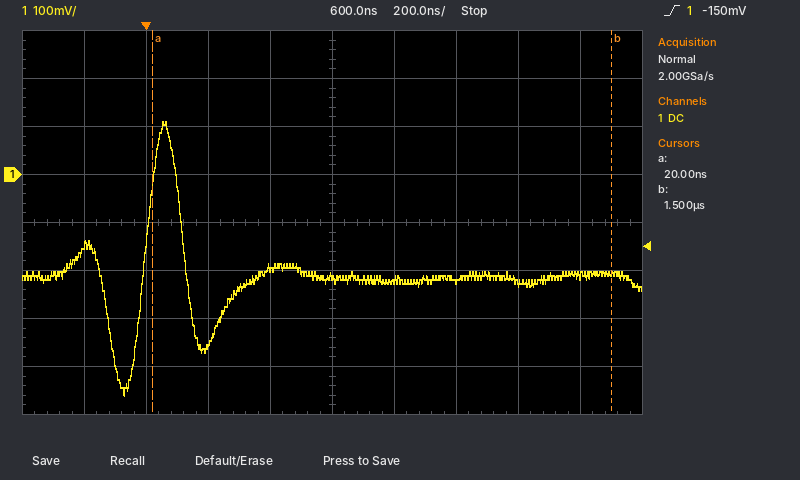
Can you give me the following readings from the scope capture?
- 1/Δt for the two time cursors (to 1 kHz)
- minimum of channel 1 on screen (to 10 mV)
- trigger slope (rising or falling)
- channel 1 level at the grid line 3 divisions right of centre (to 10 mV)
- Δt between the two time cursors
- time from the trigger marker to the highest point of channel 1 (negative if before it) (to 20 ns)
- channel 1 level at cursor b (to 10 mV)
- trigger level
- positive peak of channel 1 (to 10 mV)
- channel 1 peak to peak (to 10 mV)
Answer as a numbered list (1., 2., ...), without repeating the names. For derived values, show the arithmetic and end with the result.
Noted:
1. 1 / 1.48 µs ≈ 676 kHz
2. -460 mV
3. rising
4. -230 mV
5. 1.5 µs − (20 ns) = 1.48 µs
6. +60 ns
7. -210 mV
8. -150 mV
9. 110 mV
10. 110 mV − (-460 mV) = 570 mV
